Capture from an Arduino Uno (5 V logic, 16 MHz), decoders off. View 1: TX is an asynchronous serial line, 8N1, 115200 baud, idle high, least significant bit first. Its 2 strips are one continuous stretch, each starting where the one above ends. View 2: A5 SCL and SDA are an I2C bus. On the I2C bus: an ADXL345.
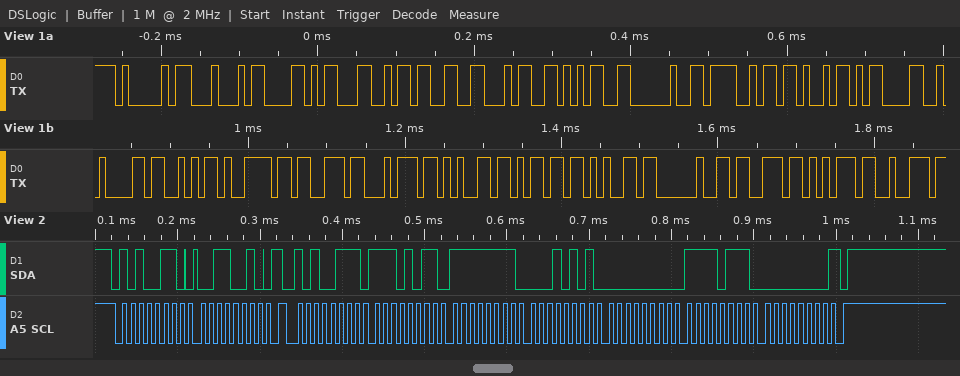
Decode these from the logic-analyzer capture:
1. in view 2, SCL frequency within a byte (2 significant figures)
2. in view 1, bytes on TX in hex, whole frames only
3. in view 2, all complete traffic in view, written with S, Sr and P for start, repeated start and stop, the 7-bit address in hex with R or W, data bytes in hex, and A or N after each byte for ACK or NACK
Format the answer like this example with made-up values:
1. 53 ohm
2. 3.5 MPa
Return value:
1. 100 kHz
2. 41 44 58 4C 33 34 35 20 4F 4B 0D 0A 53 79 73 74 65 6D 65 20 73 75 72
3. S 53W A 32 A Sr 53R A EB A FF A 15 A 00 A F7 A 00 N P
